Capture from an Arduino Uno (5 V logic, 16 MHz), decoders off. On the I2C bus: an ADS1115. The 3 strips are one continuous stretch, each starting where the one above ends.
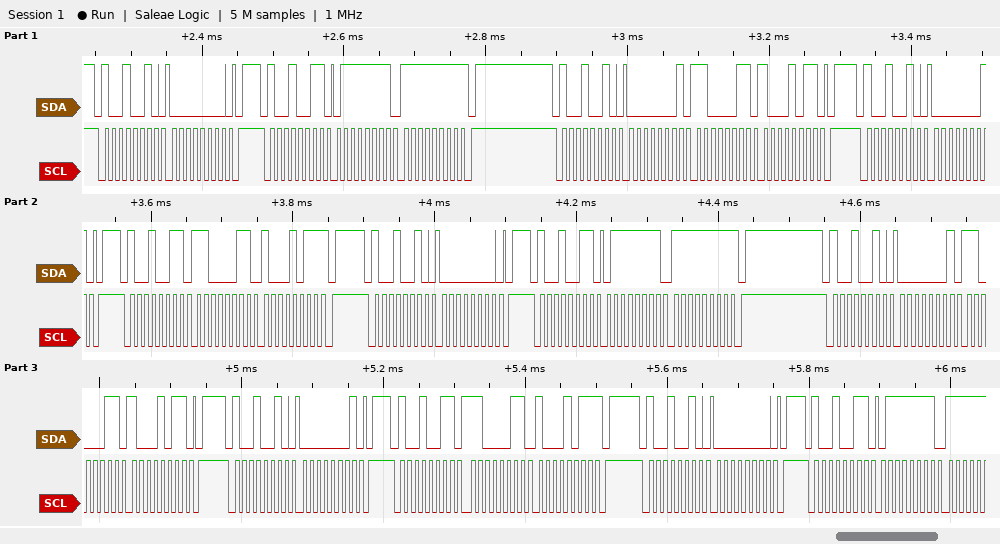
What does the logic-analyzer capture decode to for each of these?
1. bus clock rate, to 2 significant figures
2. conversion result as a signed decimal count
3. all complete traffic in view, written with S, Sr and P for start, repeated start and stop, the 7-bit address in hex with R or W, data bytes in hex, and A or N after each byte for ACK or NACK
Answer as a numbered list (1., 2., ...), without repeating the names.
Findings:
1. 100 kHz
2. 32767
3. S 49W A 00 A P S 49R A 7F A FF N P S 49W A 01 A C3 A 8B A P S 49W A 01 A P S 49R A C3 A 8B N P S 49W A 00 A P S 49R A 7F A FF N P S 49W A 01 A C3 A 8B A P S 49W A 01 A P S 49R A C3 A 8B N P S 49W A 00 A P S 49R A 7F A
